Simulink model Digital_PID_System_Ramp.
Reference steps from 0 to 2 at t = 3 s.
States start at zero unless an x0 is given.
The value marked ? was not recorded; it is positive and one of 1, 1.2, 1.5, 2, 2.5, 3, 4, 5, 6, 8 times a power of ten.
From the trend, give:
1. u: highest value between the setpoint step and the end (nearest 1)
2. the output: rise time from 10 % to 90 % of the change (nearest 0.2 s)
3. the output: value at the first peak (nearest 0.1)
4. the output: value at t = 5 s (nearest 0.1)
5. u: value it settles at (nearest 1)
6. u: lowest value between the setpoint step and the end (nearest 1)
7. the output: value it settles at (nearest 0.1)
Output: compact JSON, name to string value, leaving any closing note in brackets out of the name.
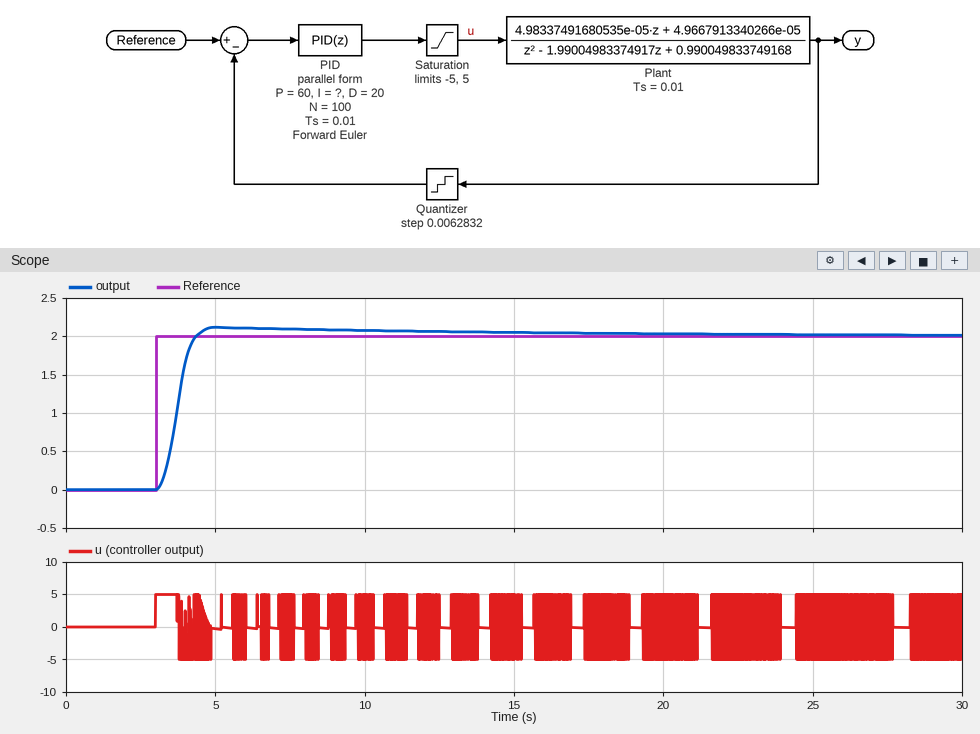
{"u: highest value between the setpoint step and the end": "5", "the output: rise time from 10 % to 90 % of the change": "0.8 s", "the output: value at the first peak": "2.1", "the output: value at t = 5 s": "2.1", "u: value it settles at": "0", "u: lowest value between the setpoint step and the end": "-5", "the output: value it settles at": "2.0"}
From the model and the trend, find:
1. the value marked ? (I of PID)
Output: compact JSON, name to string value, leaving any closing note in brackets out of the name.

{"the value marked ?": "5"}
